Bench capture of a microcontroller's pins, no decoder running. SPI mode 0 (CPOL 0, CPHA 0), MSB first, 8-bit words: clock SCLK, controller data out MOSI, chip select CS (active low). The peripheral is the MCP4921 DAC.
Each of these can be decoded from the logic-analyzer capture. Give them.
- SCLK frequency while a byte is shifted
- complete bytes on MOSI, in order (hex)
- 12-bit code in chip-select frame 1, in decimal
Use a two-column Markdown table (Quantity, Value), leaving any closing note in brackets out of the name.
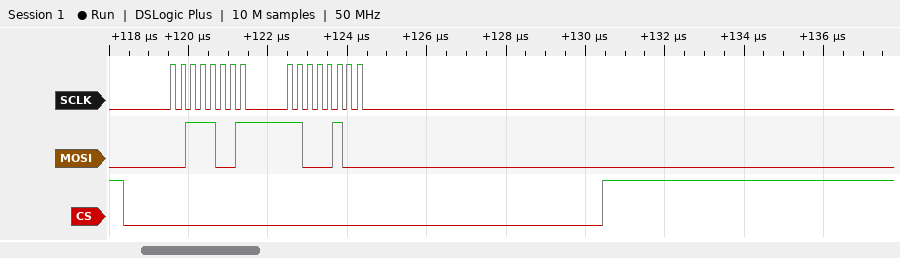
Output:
| Quantity | Value |
|---|---|
| SCLK frequency while a byte is shifted | 4 MHz |
| complete bytes on MOSI, in order | 39 C4 |
| 12-bit code in chip-select frame 1, in decimal | 2500 |
